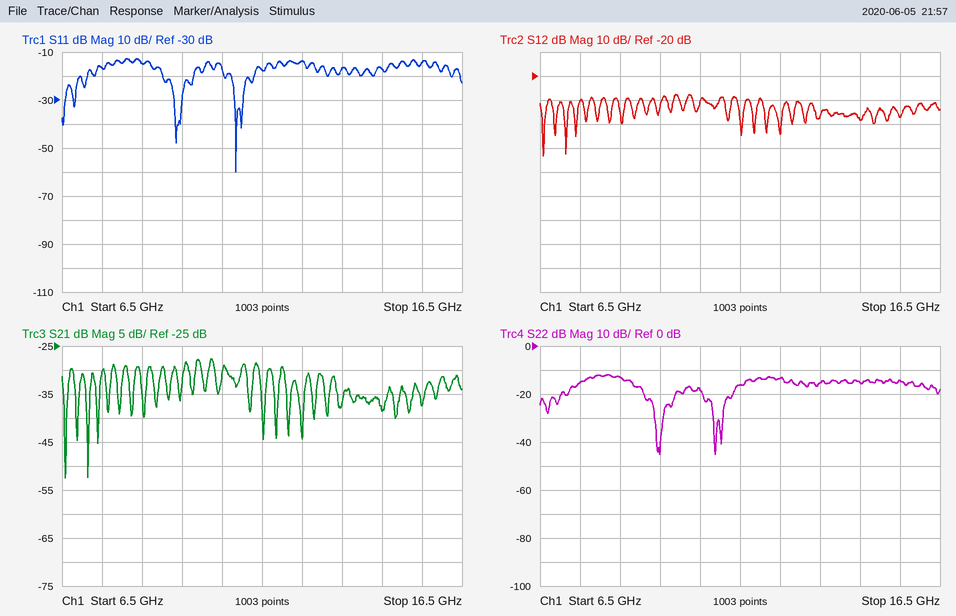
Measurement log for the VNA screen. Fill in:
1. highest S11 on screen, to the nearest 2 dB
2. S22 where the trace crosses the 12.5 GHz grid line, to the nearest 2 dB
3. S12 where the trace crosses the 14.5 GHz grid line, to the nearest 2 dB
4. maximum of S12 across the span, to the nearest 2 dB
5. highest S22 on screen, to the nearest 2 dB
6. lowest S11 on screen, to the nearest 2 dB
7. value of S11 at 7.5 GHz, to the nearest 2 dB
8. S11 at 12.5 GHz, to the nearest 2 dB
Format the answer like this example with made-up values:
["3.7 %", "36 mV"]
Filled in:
["-12 dB", "-14 dB", "-38 dB", "-28 dB", "-12 dB", "-60 dB", "-16 dB", "-14 dB"]
